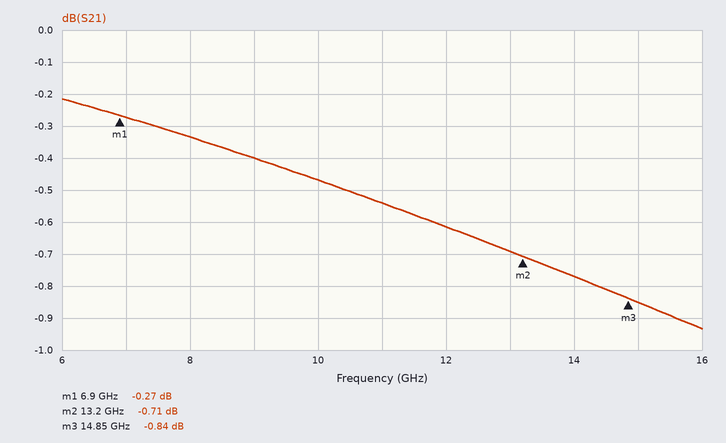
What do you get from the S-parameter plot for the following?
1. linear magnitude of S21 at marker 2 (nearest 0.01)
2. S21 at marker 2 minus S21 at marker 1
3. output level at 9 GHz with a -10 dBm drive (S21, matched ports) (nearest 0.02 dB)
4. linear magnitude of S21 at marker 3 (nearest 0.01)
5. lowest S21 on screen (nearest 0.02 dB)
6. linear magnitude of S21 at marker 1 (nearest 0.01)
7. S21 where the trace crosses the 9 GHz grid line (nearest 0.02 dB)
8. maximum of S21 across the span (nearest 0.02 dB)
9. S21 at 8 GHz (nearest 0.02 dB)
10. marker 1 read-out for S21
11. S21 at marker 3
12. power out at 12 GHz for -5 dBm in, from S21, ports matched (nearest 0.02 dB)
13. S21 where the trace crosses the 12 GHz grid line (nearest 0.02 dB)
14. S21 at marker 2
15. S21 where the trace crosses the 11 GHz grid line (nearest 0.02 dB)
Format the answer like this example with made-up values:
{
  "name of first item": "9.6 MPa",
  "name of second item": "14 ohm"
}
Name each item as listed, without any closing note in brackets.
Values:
{
  "linear magnitude of S21 at marker 2": "0.92",
  "S21 at marker 2 minus S21 at marker 1": "-0.44 dB",
  "output level at 9 GHz with a -10 dBm drive (S21, matched ports)": "-10.40 dBm",
  "linear magnitude of S21 at marker 3": "0.91",
  "lowest S21 on screen": "-0.94 dB",
  "linear magnitude of S21 at marker 1": "0.97",
  "S21 where the trace crosses the 9 GHz grid line": "-0.40 dB",
  "maximum of S21 across the span": "-0.22 dB",
  "S21 at 8 GHz": "-0.34 dB",
  "marker 1 read-out for S21": "-0.27 dB",
  "S21 at marker 3": "-0.84 dB",
  "power out at 12 GHz for -5 dBm in, from S21, ports matched": "-5.62 dBm",
  "S21 where the trace crosses the 12 GHz grid line": "-0.62 dB",
  "S21 at marker 2": "-0.71 dB",
  "S21 where the trace crosses the 11 GHz grid line": "-0.54 dB"
}
